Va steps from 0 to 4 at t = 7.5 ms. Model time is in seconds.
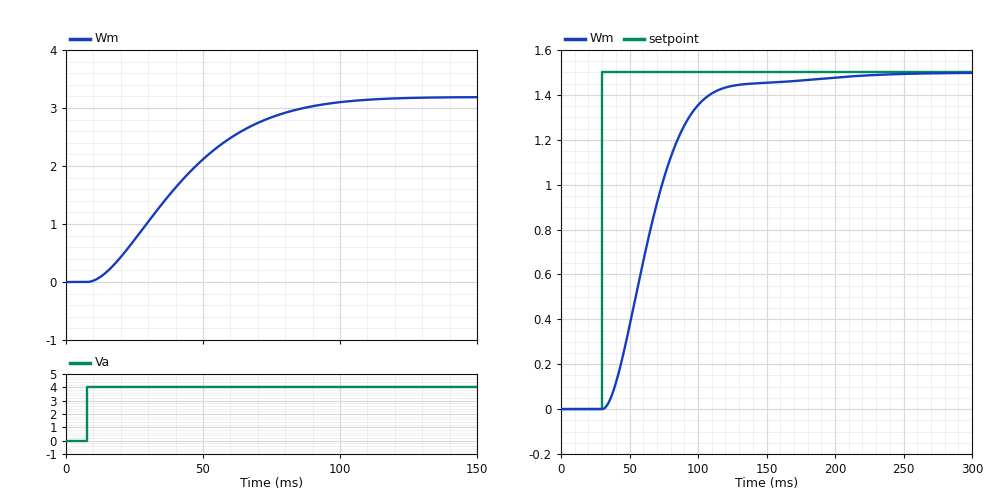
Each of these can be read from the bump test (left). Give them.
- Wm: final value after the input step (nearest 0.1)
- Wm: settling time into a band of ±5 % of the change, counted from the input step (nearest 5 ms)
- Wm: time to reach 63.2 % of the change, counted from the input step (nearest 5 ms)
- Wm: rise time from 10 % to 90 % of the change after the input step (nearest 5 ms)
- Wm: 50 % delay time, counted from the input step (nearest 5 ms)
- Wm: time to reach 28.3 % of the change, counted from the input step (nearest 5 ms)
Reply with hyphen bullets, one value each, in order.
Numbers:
- 3.2
- 80 ms
- 40 ms
- 60 ms
- 30 ms
- 20 ms
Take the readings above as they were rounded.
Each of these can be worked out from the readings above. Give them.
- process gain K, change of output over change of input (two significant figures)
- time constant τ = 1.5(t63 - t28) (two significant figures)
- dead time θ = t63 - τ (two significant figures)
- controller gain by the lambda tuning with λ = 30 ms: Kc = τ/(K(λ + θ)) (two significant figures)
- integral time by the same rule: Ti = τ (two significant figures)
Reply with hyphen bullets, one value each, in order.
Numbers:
- 0.80
- 30 ms
- 10 ms
- 0.94
- 30 ms
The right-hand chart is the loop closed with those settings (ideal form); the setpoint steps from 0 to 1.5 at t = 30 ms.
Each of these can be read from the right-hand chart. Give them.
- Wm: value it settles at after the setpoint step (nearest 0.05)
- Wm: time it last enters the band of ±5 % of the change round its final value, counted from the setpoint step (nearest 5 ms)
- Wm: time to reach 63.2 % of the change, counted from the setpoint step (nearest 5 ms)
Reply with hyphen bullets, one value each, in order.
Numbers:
- 1.50
- 85 ms
- 40 ms
